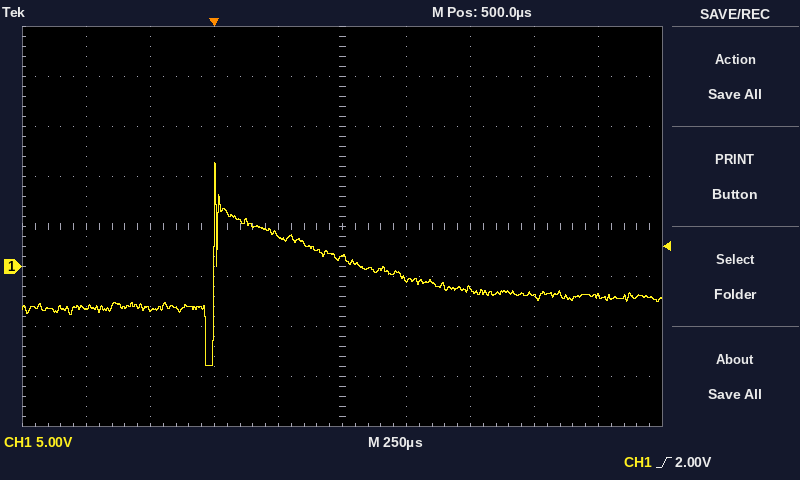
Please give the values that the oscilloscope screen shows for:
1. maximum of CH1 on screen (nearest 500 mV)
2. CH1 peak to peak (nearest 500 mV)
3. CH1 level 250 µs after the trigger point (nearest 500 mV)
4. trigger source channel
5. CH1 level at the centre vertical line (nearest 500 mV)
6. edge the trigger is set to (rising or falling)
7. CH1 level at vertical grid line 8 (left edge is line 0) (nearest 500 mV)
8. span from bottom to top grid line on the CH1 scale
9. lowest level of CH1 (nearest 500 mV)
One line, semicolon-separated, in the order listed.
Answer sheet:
10.5 V; 20.5 V; 3.0 V; CH1; 1.0 V; rising; -3.0 V; 40 V; -10.0 V
